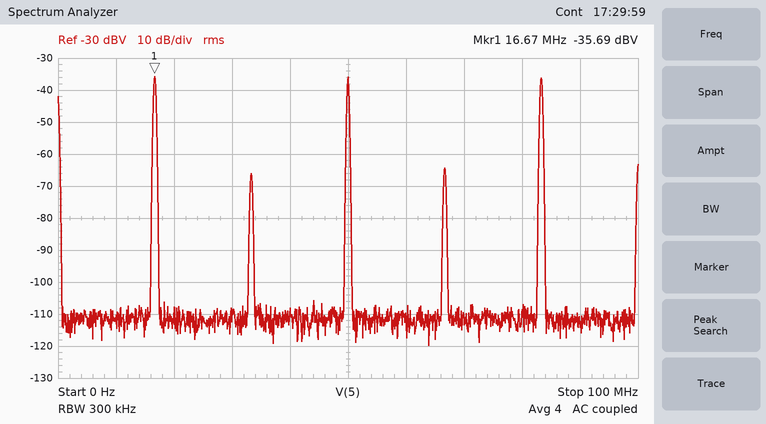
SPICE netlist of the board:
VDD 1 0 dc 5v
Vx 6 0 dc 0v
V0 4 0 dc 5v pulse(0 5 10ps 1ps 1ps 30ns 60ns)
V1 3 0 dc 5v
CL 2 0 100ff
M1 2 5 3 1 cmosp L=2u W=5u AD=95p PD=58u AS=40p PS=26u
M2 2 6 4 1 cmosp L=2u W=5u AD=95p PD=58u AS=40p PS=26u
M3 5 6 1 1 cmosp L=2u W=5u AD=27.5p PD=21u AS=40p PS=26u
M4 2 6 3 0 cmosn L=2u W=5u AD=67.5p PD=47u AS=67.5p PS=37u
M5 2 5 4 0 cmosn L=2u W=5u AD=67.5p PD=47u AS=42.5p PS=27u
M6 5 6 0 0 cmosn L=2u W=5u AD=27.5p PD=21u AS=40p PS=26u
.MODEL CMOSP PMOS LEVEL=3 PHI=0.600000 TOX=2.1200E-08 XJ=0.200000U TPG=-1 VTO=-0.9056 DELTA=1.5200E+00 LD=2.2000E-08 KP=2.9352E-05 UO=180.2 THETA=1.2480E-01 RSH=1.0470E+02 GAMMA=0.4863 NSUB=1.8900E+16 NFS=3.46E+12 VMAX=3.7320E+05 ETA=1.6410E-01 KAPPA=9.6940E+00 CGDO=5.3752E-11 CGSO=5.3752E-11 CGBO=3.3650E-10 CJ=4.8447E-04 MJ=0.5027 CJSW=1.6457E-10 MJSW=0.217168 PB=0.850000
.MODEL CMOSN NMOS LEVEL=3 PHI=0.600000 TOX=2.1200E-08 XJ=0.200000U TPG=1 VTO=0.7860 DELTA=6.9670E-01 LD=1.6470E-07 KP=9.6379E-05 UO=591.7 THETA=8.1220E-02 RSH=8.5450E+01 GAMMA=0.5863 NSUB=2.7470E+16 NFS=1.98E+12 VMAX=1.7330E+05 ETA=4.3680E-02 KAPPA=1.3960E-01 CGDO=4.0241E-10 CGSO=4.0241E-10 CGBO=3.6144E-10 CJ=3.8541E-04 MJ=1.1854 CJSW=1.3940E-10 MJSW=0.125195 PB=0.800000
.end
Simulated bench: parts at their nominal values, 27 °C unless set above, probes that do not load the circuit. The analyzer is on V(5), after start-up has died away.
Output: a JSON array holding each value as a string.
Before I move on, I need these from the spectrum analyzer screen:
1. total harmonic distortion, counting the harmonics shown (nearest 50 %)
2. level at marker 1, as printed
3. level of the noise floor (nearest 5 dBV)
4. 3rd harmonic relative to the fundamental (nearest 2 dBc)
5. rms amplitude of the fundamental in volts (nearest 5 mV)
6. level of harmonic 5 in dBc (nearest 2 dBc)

["150 %", "-35.69 dBV", "-110 dBV", "0 dBc", "15 mV", "0 dBc"]
